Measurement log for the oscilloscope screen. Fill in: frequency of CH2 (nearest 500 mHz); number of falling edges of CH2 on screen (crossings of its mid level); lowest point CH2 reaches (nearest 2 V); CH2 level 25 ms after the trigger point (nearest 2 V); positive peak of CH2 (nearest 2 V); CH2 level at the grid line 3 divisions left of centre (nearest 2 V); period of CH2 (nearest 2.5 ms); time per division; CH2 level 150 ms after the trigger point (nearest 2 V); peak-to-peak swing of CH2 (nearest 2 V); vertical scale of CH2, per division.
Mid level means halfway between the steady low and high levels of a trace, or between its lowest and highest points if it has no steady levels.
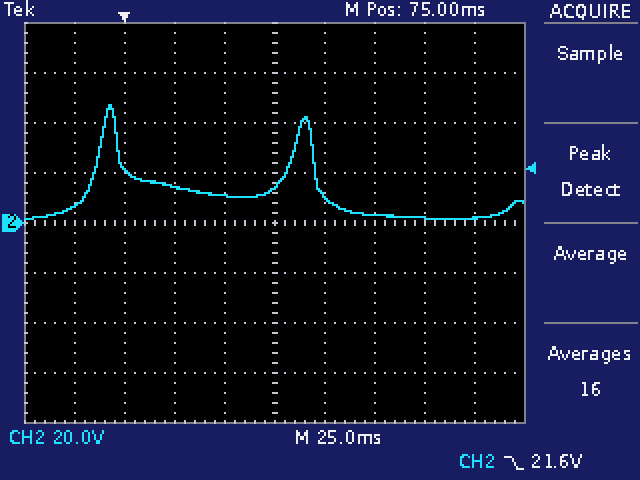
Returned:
10.5 Hz
2
2 V
14 V
48 V
22 V
97.5 ms
25 ms
2 V
46 V
20 V
